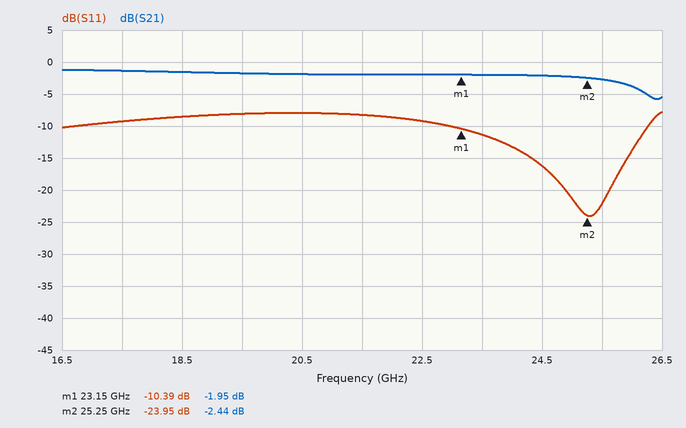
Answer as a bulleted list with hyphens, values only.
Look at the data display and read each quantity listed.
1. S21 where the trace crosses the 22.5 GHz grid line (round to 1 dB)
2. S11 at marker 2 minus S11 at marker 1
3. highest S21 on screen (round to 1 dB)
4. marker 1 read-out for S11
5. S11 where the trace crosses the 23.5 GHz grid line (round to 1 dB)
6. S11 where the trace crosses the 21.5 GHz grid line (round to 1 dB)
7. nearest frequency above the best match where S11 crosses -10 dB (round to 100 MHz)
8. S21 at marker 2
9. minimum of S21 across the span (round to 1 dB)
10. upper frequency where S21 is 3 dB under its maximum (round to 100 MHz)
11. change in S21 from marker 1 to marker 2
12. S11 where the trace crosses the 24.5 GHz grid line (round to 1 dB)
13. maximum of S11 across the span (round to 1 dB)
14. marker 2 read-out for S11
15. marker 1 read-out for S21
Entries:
- -2 dB
- -13.56 dB
- -1 dB
- -10.39 dB
- -11 dB
- -8 dB
- 26.3 GHz
- -2.44 dB
- -6 dB
- 26.1 GHz
- -0.49 dB
- -16 dB
- -8 dB
- -23.95 dB
- -1.95 dB
